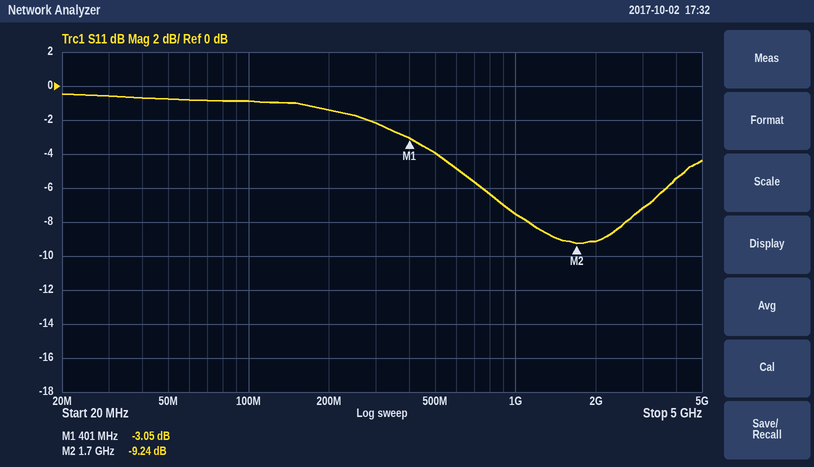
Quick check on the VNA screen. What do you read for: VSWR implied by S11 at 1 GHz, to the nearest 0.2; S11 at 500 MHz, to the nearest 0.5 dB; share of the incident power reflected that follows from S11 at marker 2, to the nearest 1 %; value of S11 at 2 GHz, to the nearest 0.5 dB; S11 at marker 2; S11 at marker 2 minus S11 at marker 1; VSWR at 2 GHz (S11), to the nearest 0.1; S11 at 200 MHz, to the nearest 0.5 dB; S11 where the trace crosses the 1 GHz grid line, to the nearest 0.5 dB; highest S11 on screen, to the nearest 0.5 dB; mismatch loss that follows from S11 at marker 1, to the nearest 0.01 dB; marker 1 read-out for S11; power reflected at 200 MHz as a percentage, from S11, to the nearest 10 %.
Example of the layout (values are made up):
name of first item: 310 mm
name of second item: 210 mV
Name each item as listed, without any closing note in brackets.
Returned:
VSWR implied by S11 at 1 GHz, to the nearest 0.2: 2.4
S11 at 500 MHz, to the nearest 0.5 dB: -4.0 dB
share of the incident power reflected that follows from S11 at marker 2, to the nearest 1 %: 12 %
value of S11 at 2 GHz, to the nearest 0.5 dB: -9.0 dB
S11 at marker 2: -9.24 dB
S11 at marker 2 minus S11 at marker 1: -6.19 dB
VSWR at 2 GHz (S11), to the nearest 0.1: 2.1
S11 at 200 MHz, to the nearest 0.5 dB: -1.5 dB
S11 where the trace crosses the 1 GHz grid line, to the nearest 0.5 dB: -7.5 dB
highest S11 on screen, to the nearest 0.5 dB: -0.5 dB
mismatch loss that follows from S11 at marker 1, to the nearest 0.01 dB: 2.97 dB
marker 1 read-out for S11: -3.05 dB
power reflected at 200 MHz as a percentage, from S11, to the nearest 10 %: 70 %
